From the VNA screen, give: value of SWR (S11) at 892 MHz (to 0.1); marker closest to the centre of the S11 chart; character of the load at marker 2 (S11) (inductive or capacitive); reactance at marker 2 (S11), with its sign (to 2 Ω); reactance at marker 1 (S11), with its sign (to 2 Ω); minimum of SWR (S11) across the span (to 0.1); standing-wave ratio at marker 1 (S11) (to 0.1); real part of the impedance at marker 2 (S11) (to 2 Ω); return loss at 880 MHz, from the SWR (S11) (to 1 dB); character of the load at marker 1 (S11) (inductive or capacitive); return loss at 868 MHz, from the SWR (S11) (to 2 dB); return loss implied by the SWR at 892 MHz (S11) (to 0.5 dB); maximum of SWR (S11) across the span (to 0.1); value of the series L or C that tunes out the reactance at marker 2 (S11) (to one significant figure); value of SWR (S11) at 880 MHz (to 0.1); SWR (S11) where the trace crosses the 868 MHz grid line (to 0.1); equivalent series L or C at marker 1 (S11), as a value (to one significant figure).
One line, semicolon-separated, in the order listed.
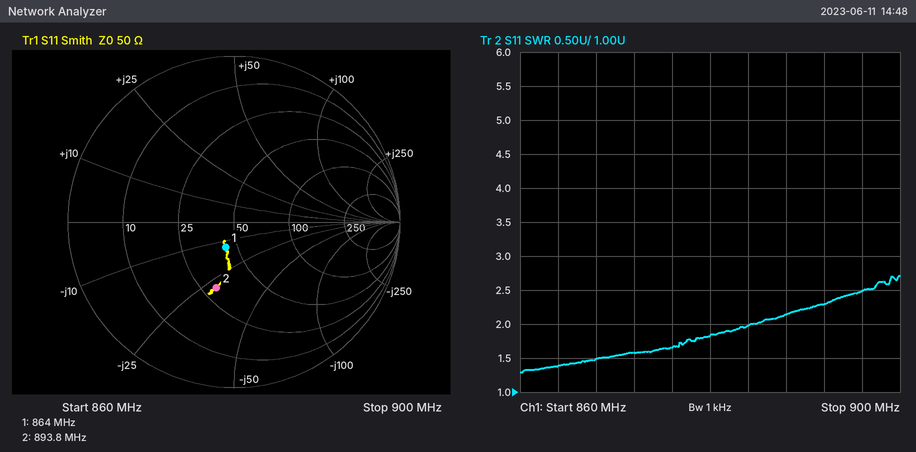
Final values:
2.3; marker 1; capacitive; -28 Ω; -14 Ω; 1.3; 1.4; 30 Ω; 11 dB; capacitive; 14 dB; 8.0 dB; 2.7; 5 nH; 1.8; 1.5; 10 pF
